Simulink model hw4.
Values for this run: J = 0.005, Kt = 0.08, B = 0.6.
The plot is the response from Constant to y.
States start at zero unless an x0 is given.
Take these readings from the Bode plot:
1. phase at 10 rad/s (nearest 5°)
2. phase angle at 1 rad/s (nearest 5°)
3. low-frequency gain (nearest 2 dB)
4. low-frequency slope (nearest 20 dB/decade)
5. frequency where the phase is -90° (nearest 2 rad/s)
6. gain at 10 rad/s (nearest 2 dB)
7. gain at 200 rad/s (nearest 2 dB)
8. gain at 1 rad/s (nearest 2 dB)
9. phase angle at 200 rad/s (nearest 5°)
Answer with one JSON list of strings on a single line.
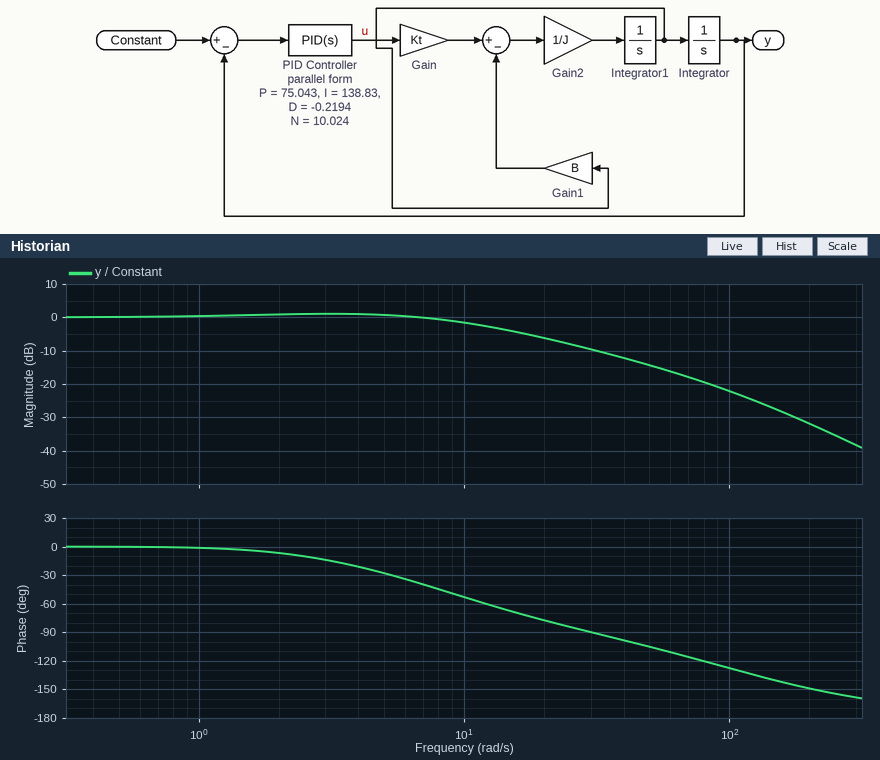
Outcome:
["-55°", "0°", "0 dB", "0 dB/decade", "30 rad/s", "-2 dB", "-32 dB", "0 dB", "-150°"]
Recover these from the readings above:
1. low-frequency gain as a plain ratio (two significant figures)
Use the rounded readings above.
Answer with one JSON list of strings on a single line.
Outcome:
["1.0"]
